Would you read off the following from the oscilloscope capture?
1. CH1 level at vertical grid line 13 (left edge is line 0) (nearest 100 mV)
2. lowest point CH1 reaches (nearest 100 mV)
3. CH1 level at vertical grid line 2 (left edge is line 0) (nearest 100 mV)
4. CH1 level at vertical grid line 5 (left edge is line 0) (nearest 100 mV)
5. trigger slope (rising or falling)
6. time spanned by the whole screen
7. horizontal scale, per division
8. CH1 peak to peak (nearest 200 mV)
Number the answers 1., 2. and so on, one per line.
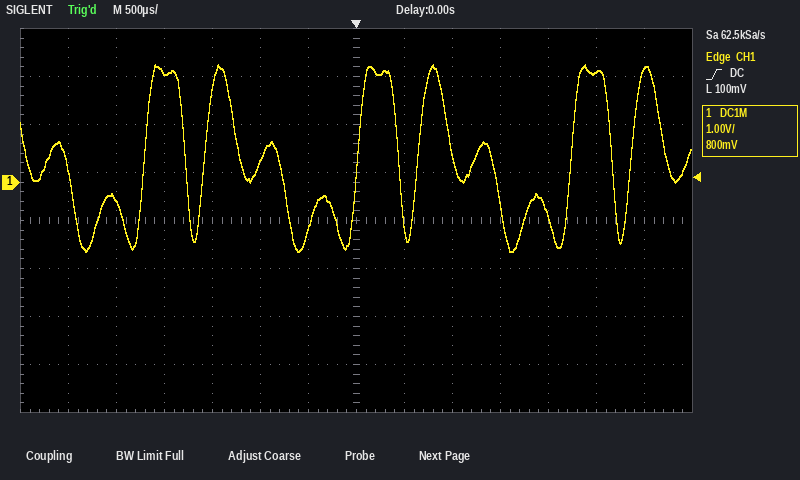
1. 2.3 V
2. -1.4 V
3. -400 mV
4. 400 mV
5. rising
6. 7 ms
7. 500 µs
8. 3.8 V
